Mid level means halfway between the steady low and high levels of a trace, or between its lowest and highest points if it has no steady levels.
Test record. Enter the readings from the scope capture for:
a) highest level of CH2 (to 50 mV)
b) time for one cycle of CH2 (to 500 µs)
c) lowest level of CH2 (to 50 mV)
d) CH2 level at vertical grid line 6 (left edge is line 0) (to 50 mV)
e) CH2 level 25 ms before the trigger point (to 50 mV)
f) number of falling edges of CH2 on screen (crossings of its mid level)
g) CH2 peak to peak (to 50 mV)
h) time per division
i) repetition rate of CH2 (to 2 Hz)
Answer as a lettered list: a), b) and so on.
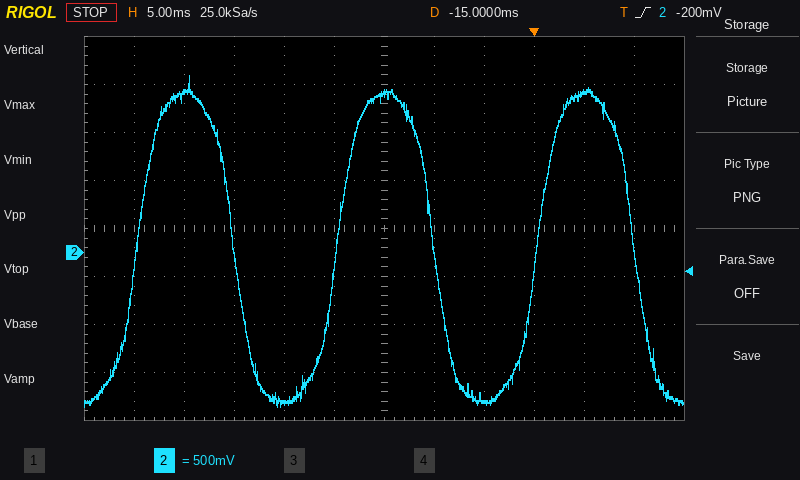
a) 1.85 V
b) 20.0 ms
c) -1.60 V
d) 1.65 V
e) -1.55 V
f) 3
g) 3.45 V
h) 5 ms
i) 50 Hz
